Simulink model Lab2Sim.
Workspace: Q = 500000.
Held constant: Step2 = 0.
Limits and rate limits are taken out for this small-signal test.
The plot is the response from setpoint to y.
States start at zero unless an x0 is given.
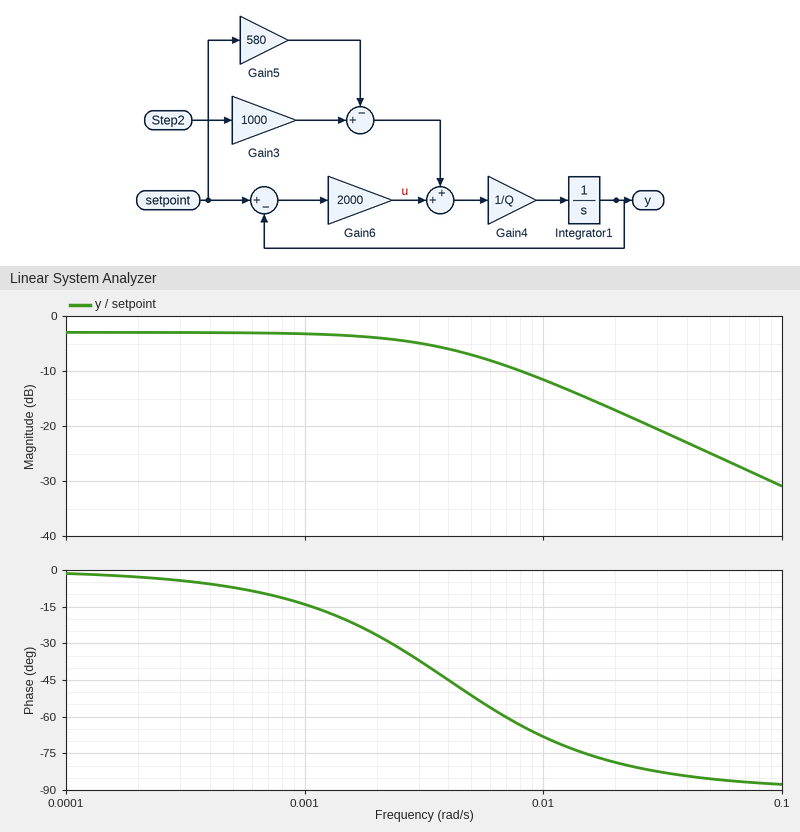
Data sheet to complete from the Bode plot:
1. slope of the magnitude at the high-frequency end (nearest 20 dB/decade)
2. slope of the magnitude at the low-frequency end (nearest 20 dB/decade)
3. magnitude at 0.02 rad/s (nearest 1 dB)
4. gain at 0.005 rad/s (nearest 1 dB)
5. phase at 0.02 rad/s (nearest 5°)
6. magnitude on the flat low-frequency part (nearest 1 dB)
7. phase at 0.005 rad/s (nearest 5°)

-20 dB/decade
0 dB/decade
-17 dB
-7 dB
-80°
-3 dB
-50°
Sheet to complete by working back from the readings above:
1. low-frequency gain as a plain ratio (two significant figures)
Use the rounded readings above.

0.71
